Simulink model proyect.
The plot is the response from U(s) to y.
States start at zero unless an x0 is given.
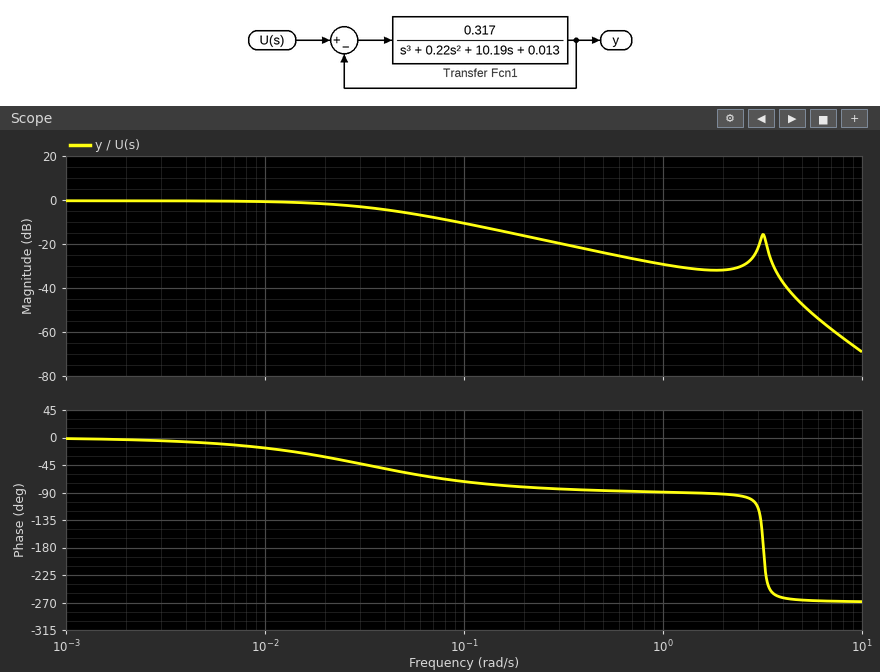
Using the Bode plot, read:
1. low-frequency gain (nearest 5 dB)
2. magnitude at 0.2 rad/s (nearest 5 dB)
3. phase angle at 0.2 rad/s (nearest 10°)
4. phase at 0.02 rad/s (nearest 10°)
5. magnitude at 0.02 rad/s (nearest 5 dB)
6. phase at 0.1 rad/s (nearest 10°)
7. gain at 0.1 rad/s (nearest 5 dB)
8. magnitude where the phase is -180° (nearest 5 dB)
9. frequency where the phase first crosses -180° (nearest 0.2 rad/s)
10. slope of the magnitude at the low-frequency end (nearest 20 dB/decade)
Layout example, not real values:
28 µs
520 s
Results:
0 dB
-15 dB
-80°
-30°
0 dB
-70°
-10 dB
-15 dB
3.2 rad/s
0 dB/decade
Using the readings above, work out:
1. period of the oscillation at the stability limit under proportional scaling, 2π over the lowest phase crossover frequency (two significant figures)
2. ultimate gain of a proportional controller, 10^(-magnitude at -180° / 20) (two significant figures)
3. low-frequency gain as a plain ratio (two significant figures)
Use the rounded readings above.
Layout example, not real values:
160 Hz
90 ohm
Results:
2.0 s
5.6
1.0
